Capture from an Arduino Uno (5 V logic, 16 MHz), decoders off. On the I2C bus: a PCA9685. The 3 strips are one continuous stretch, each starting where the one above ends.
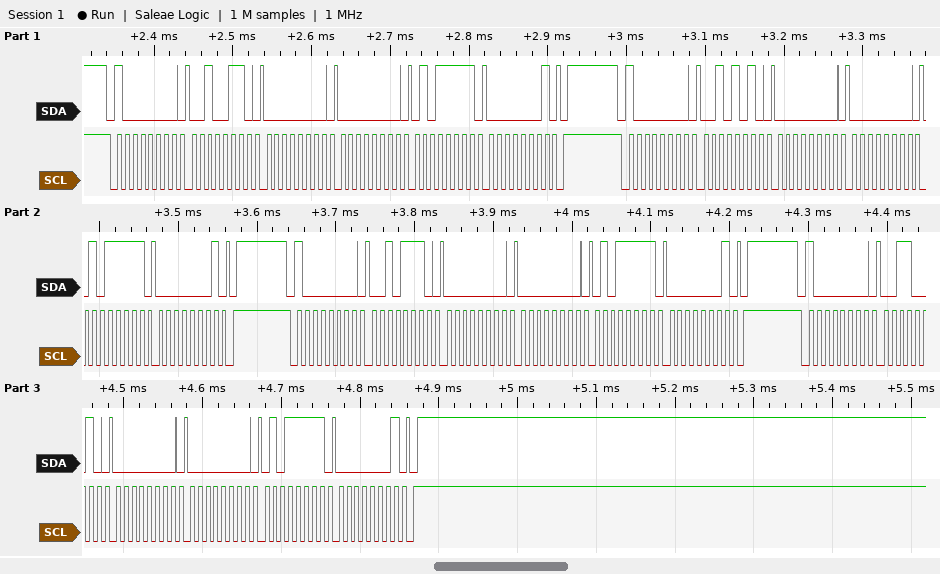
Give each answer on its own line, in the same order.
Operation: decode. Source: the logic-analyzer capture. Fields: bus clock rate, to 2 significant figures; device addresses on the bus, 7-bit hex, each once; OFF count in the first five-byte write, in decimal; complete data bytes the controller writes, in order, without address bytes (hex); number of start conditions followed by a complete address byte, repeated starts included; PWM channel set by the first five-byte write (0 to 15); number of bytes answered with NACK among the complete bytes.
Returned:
100 kHz
0x40
351
26 00 00 5F 01 2A 00 00 5F 01 2E 00 00 5F 01 32 00 00 5F 01
4
8
0
